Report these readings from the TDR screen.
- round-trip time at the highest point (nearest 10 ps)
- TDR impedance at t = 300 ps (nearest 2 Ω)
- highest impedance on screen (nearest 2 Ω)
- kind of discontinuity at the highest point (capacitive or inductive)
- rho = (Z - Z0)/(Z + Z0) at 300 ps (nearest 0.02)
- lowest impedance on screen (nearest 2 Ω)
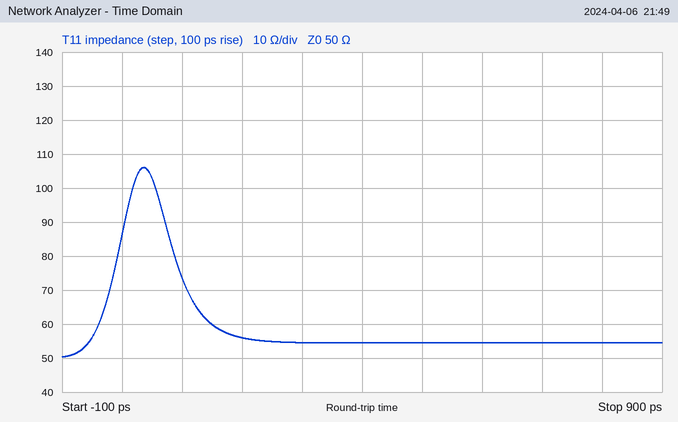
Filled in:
40 ps
54 Ω
106 Ω
inductive
+0.04
50 Ω
